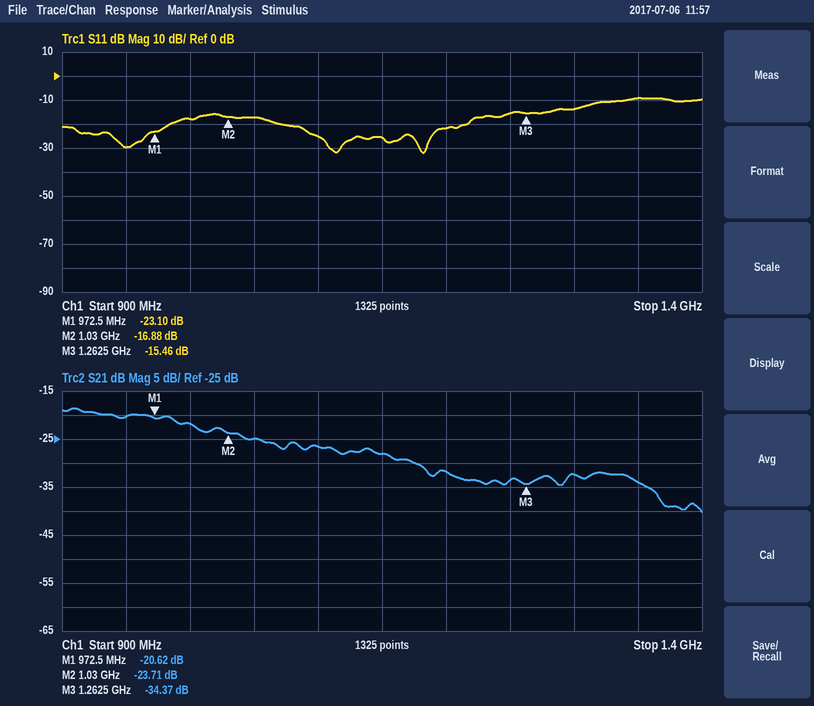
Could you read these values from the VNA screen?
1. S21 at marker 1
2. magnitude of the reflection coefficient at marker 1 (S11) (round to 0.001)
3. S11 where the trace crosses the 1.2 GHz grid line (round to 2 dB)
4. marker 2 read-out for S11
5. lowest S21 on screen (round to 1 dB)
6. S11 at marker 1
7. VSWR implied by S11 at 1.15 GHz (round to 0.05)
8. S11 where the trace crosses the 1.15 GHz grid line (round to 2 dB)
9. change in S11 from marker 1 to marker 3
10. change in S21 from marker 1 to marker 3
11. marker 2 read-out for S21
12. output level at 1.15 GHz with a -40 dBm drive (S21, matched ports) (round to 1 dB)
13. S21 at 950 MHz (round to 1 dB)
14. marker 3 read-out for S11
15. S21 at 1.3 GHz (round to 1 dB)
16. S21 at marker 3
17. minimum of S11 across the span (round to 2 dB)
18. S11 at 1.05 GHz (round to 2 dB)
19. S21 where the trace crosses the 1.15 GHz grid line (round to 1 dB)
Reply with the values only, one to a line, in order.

-20.62 dB
0.070
-22 dB
-16.88 dB
-40 dB
-23.10 dB
1.10
-26 dB
7.64 dB
-13.75 dB
-23.71 dB
-68 dBm
-20 dB
-15.46 dB
-32 dB
-34.37 dB
-32 dB
-18 dB
-28 dB
